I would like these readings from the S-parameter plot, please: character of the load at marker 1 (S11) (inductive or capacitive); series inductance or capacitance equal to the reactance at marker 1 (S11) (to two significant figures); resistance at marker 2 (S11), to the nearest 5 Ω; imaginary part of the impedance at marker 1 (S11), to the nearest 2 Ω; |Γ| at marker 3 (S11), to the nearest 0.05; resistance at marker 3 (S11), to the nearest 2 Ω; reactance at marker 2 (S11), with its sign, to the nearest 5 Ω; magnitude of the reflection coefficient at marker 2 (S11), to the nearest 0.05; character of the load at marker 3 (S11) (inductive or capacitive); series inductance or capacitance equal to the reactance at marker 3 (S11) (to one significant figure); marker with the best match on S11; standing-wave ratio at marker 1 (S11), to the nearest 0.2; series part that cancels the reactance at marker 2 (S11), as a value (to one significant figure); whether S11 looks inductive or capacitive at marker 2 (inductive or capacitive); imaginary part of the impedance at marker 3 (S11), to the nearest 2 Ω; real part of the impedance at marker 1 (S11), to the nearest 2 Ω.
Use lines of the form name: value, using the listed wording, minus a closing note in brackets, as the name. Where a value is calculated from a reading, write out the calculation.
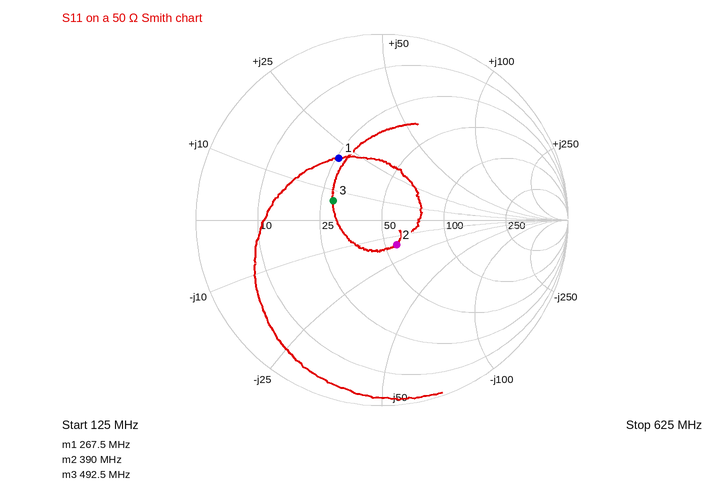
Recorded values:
character of the load at marker 1 (S11): inductive
series inductance or capacitance equal to the reactance at marker 1 (S11): L = 20 Ω/(2π × 267.5 MHz) ≈ 12 nH
resistance at marker 2 (S11), to the nearest 5 Ω: 55 Ω
imaginary part of the impedance at marker 1 (S11), to the nearest 2 Ω: +20 Ω
|Γ| at marker 3 (S11), to the nearest 0.05: 0.30
resistance at marker 3 (S11), to the nearest 2 Ω: 28 Ω
reactance at marker 2 (S11), with its sign, to the nearest 5 Ω: -15 Ω
magnitude of the reflection coefficient at marker 2 (S11), to the nearest 0.05: 0.15
character of the load at marker 3 (S11): inductive
series inductance or capacitance equal to the reactance at marker 3 (S11): L = 6 Ω/(2π × 492.5 MHz) ≈ 2 nH
marker with the best match on S11: marker 2
standing-wave ratio at marker 1 (S11), to the nearest 0.2: 2.4
series part that cancels the reactance at marker 2 (S11), as a value: L = 15 Ω/(2π × 390 MHz) ≈ 6 nH
whether S11 looks inductive or capacitive at marker 2: capacitive
imaginary part of the impedance at marker 3 (S11), to the nearest 2 Ω: +6 Ω
real part of the impedance at marker 1 (S11), to the nearest 2 Ω: 26 Ω
